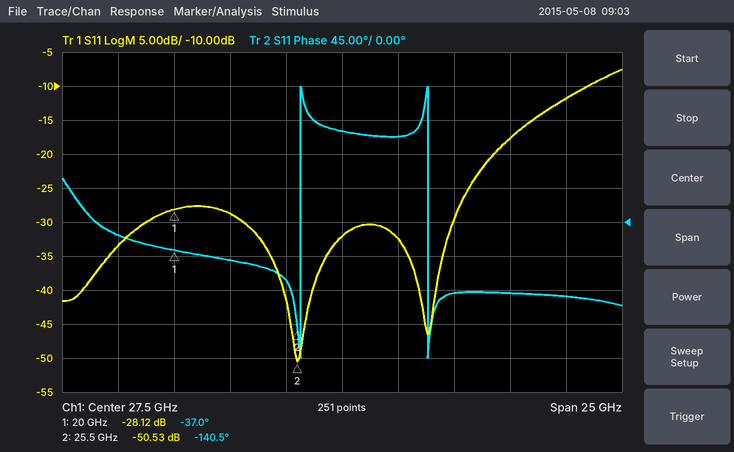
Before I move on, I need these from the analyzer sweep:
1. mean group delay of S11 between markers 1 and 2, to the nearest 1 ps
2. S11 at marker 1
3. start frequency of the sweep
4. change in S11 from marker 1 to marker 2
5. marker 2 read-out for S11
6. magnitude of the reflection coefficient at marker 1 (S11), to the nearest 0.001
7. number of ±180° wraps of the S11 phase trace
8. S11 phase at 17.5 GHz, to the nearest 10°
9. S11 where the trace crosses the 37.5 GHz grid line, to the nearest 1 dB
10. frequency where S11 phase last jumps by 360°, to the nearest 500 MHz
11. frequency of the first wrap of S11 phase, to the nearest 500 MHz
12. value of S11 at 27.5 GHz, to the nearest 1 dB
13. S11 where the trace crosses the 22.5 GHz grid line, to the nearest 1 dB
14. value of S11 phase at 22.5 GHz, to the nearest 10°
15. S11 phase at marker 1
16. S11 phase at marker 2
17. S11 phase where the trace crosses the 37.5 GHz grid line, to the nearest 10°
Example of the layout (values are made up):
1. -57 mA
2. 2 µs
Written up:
1. 52 ps
2. -28.12 dB
3. 15 GHz
4. -22.41 dB
5. -50.53 dB
6. 0.039
7. 2
8. -20°
9. -12 dB
10. 31.5 GHz
11. 25.5 GHz
12. -32 dB
13. -29 dB
14. -50°
15. -37.0°
16. -140.5°
17. -100°
